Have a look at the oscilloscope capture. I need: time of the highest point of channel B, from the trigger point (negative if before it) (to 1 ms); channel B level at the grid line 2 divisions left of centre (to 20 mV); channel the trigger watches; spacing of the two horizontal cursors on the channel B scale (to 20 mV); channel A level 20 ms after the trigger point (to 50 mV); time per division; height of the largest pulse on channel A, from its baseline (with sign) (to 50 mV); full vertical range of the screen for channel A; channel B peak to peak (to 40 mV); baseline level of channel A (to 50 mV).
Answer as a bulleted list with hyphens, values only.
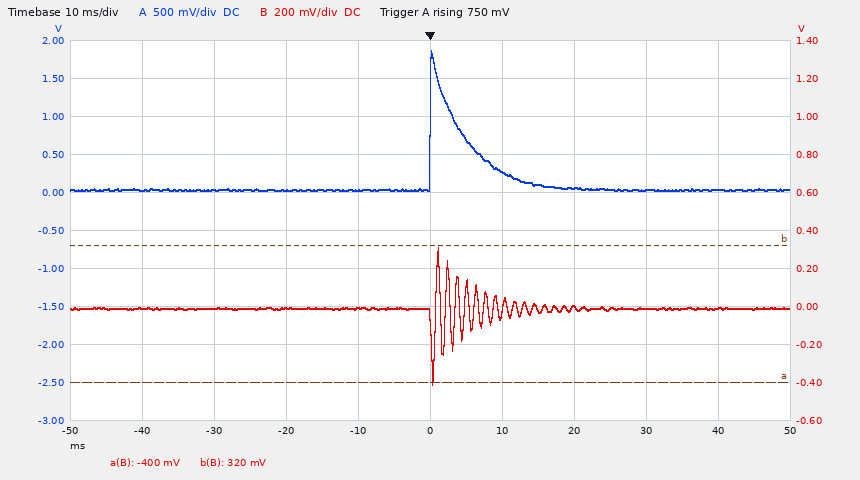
- +1 ms
- 0 mV
- channel A
- 720 mV
- 50 mV
- 10 ms
- +1.85 V
- 5 V
- 720 mV
- 50 mV
